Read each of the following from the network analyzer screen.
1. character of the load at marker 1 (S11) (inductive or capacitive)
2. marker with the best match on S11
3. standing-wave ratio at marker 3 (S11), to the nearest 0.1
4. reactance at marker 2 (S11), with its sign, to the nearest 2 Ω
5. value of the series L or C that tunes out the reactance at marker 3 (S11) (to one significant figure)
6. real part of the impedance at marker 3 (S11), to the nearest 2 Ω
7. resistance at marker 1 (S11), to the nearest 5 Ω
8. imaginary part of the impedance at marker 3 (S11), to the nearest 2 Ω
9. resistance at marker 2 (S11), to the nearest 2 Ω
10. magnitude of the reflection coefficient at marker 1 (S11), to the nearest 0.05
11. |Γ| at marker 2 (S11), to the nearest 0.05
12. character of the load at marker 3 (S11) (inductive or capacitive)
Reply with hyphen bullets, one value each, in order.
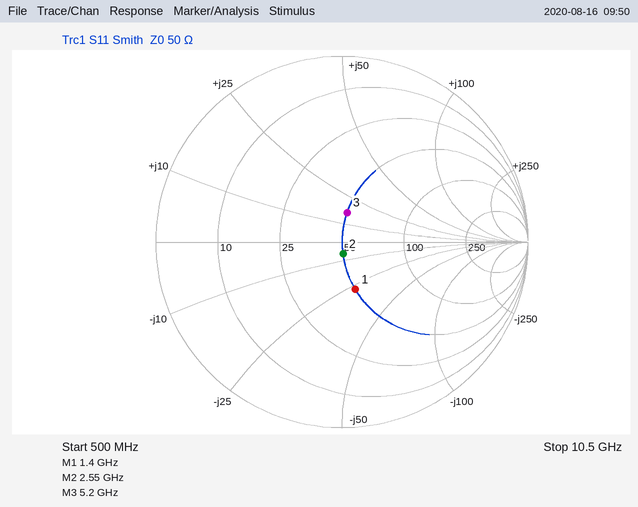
- capacitive
- marker 2
- 1.4
- -6 Ω
- 2 pF
- 50 Ω
- 50 Ω
- +16 Ω
- 50 Ω
- 0.25
- 0.05
- inductive
